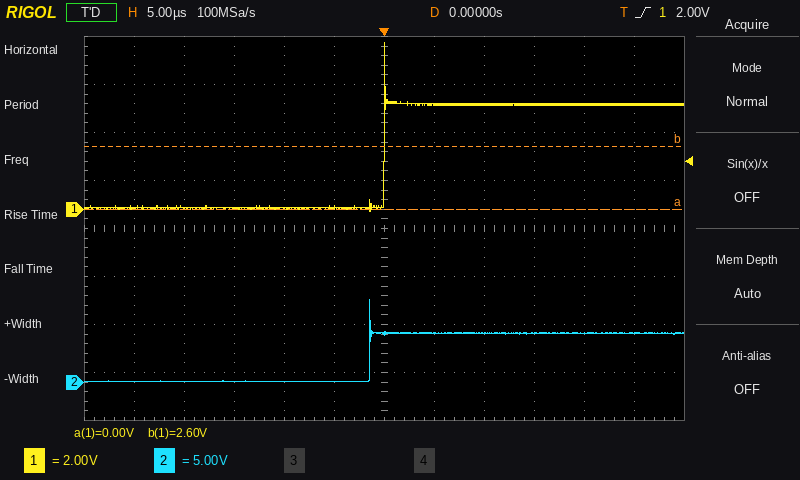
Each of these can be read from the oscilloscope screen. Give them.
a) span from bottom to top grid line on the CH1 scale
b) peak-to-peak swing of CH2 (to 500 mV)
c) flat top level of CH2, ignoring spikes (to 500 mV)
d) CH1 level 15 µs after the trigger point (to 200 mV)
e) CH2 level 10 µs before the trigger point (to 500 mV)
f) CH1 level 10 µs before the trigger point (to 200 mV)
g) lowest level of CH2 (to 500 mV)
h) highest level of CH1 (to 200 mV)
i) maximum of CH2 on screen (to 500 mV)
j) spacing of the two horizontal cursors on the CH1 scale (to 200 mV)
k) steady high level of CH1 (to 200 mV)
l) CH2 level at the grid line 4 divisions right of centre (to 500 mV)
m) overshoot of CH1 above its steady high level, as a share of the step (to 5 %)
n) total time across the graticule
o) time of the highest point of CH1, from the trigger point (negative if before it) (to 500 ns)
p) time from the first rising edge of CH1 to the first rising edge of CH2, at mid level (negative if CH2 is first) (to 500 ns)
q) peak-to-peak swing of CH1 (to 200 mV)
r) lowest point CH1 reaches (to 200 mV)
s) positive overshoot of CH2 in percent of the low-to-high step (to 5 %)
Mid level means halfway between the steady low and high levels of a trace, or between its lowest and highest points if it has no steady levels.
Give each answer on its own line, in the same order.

16 V
8.5 V
5.0 V
4.4 V
0.0 V
0.0 V
0.0 V
7.0 V
8.5 V
2.6 V
4.4 V
5.0 V
60 %
60 µs
0.0 µs
-1.5 µs
7.0 V
0.0 V
70 %
